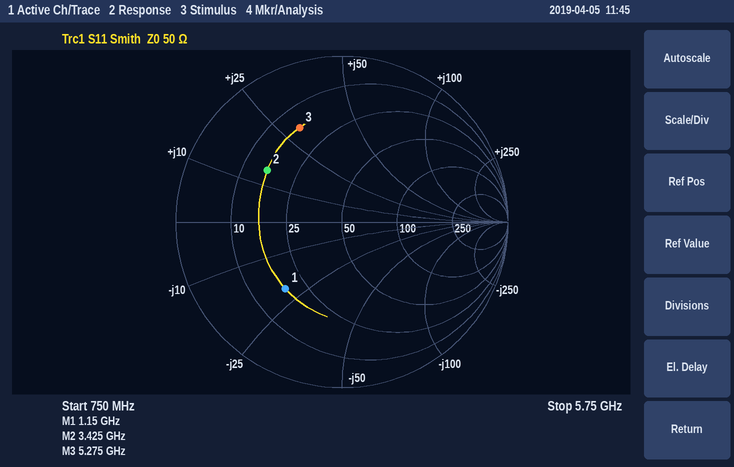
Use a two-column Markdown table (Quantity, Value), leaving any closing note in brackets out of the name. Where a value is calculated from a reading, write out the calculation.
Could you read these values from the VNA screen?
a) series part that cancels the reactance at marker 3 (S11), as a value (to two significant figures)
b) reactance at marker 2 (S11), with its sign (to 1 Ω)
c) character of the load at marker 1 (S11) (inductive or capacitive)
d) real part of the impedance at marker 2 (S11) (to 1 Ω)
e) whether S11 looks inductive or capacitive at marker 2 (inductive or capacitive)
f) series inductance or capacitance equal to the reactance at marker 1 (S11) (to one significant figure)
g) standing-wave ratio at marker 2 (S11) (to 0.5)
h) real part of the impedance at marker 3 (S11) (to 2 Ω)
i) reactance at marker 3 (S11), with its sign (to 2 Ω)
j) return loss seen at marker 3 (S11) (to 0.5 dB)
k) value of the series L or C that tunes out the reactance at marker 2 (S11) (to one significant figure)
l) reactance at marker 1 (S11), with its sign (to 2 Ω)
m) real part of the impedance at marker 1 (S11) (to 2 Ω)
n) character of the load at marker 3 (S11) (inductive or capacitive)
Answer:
| Quantity | Value |
|---|---|
| series part that cancels the reactance at marker 3 (S11), as a value | C = 1/(2π × 5.275 GHz × 30 Ω) ≈ 1.0 pF |
| reactance at marker 2 (S11), with its sign | +14 Ω |
| character of the load at marker 1 (S11) | capacitive |
| real part of the impedance at marker 2 (S11) | 16 Ω |
| whether S11 looks inductive or capacitive at marker 2 | inductive |
| series inductance or capacitance equal to the reactance at marker 1 (S11) | C = 1/(2π × 1.15 GHz × 20 Ω) ≈ 7 pF |
| standing-wave ratio at marker 2 (S11) | 3.5 |
| real part of the impedance at marker 3 (S11) | 16 Ω |
| reactance at marker 3 (S11), with its sign | +30 Ω |
| return loss seen at marker 3 (S11) | 4.0 dB |
| value of the series L or C that tunes out the reactance at marker 2 (S11) | C = 1/(2π × 3.425 GHz × 14 Ω) ≈ 3 pF |
| reactance at marker 1 (S11), with its sign | -20 Ω |
| real part of the impedance at marker 1 (S11) | 18 Ω |
| character of the load at marker 3 (S11) | inductive |
